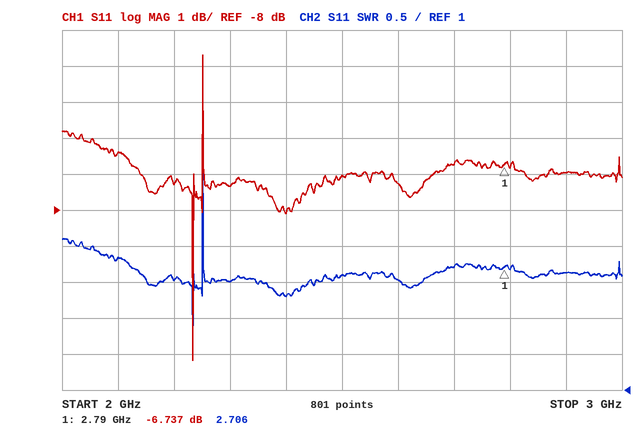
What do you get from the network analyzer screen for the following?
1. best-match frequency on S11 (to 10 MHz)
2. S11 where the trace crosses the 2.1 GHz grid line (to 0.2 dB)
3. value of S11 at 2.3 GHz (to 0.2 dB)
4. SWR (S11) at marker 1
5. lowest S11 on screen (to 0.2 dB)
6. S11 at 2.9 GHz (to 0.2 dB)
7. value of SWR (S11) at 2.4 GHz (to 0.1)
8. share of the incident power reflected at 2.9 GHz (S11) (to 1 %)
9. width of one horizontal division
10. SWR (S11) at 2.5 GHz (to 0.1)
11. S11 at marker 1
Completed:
2.23 GHz
-6.4 dB
-7.4 dB
2.706
-12.2 dB
-7.0 dB
2.3
20 %
100 MHz
2.6
-6.737 dB
